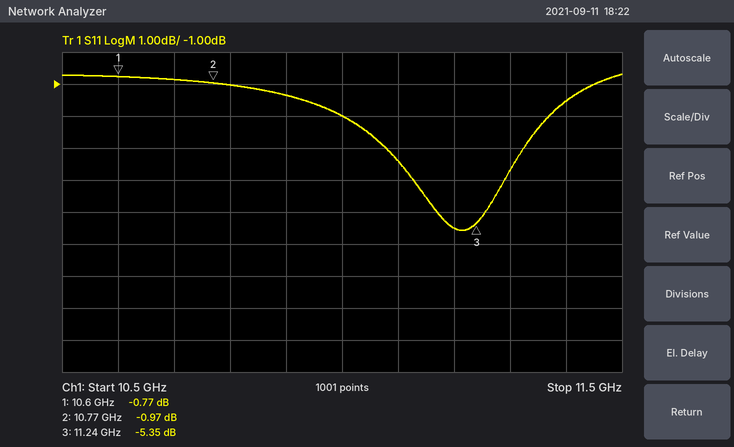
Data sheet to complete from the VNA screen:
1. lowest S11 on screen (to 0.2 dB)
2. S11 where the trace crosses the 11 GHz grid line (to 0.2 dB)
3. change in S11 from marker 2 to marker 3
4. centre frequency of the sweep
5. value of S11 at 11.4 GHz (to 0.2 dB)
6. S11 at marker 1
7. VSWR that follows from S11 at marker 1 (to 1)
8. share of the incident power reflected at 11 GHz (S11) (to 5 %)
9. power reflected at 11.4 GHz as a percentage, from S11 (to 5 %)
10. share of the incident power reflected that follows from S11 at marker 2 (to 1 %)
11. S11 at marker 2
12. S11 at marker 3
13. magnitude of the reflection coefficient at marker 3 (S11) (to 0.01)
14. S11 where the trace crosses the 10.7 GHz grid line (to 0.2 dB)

-5.6 dB
-2.0 dB
-4.38 dB
11 GHz
-1.6 dB
-0.77 dB
23
65 %
70 %
80 %
-0.97 dB
-5.35 dB
0.54
-0.8 dB
